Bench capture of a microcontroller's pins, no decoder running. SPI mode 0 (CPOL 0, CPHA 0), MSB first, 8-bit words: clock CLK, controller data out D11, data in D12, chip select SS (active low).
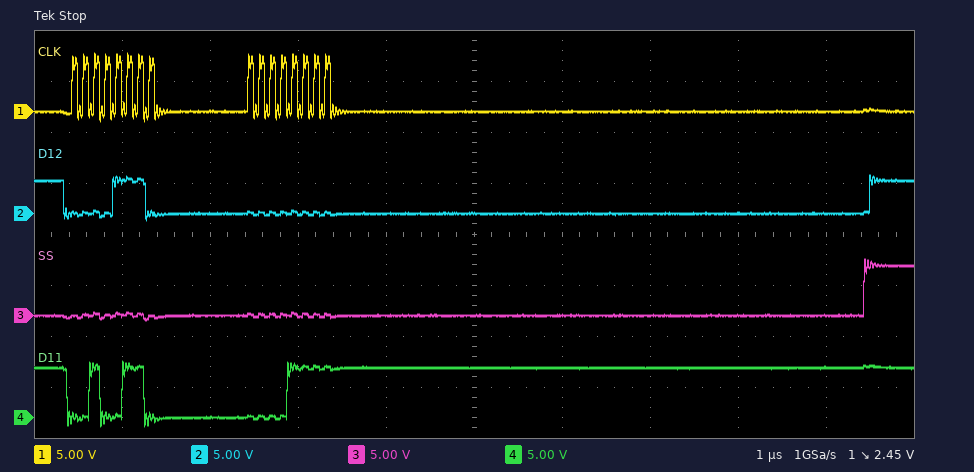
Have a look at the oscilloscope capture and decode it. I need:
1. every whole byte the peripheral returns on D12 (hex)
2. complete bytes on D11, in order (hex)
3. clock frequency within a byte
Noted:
0E 00
26 0F
8 MHz
